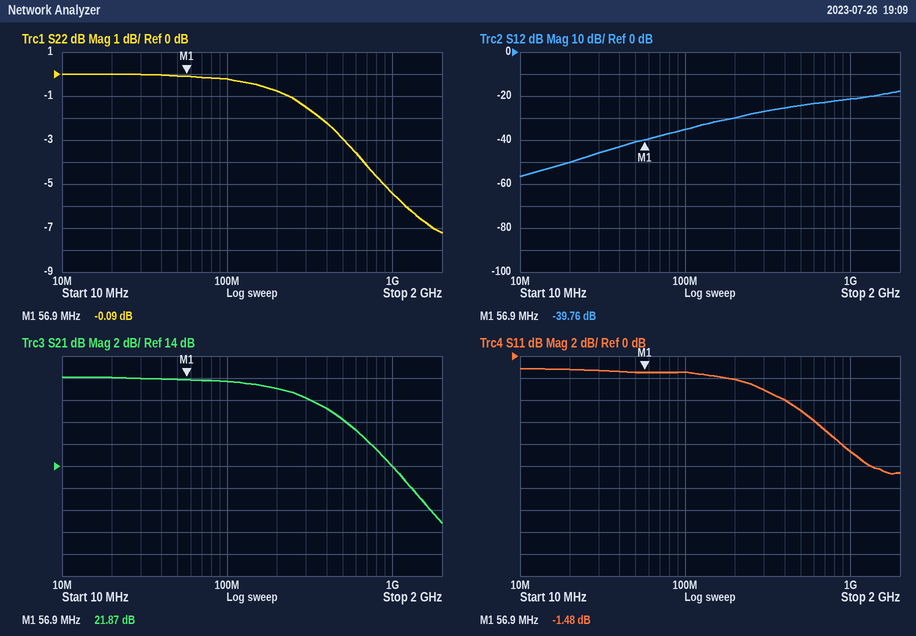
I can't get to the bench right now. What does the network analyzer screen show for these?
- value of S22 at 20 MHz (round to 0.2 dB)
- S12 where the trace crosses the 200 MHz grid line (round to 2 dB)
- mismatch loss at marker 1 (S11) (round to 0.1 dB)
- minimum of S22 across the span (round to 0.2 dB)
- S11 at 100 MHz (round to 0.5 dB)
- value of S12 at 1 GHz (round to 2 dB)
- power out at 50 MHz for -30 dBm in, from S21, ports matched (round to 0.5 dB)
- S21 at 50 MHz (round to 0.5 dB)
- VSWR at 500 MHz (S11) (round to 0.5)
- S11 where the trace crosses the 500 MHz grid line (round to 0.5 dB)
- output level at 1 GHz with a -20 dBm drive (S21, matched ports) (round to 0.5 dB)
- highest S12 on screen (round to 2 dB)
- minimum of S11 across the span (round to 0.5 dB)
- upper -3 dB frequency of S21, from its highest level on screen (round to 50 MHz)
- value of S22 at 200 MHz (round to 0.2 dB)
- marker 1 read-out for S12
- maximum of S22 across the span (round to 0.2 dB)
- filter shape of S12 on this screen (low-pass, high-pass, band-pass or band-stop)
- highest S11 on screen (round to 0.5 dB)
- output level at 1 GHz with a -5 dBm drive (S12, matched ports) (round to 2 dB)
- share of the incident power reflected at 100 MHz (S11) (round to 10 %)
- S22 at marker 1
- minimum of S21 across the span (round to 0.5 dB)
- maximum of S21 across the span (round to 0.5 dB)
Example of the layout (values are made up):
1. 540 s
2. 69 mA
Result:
1. 0.0 dB
2. -30 dB
3. 5.4 dB
4. -7.2 dB
5. -1.5 dB
6. -22 dB
7. -8.0 dBm
8. 22.0 dB
9. 3.5
10. -5.0 dB
11. -6.0 dBm
12. -18 dB
13. -10.5 dB
14. 400 MHz
15. -0.8 dB
16. -39.76 dB
17. 0.0 dB
18. high-pass
19. -1.0 dB
20. -26 dBm
21. 70 %
22. -0.09 dB
23. 9.0 dB
24. 22.0 dB
